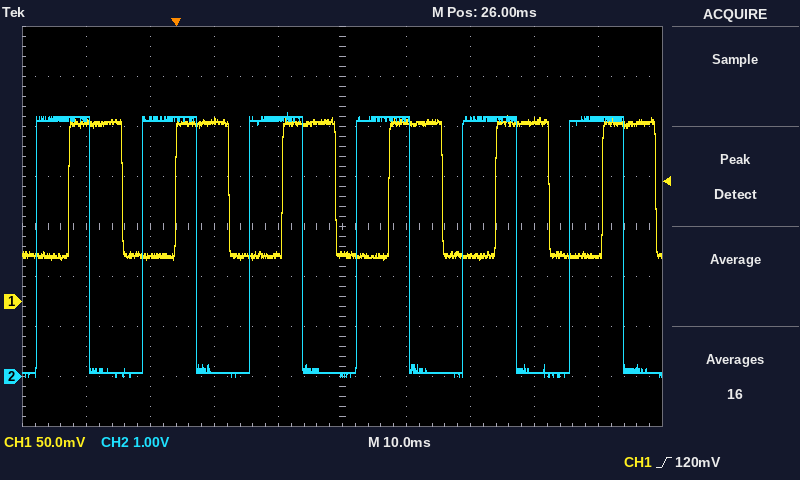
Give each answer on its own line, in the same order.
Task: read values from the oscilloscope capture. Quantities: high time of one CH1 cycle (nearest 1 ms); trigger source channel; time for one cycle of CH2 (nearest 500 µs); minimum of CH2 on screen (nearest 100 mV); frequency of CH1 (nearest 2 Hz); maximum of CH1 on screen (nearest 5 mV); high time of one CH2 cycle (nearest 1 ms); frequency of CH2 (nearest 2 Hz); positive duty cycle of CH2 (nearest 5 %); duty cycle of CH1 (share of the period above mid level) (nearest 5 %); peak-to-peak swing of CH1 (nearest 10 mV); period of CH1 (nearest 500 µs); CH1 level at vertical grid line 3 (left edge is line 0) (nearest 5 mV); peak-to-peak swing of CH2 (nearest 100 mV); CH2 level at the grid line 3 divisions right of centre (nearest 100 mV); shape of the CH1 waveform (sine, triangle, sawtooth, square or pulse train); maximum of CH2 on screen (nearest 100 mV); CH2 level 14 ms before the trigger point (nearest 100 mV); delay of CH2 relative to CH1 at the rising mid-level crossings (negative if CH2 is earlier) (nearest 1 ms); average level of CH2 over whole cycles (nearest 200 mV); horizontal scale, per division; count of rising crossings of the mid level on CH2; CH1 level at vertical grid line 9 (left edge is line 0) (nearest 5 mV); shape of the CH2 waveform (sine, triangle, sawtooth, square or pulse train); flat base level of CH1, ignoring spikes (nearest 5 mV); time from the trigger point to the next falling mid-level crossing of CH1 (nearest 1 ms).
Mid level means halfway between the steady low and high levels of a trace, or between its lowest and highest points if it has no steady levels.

8 ms
CH1
16.5 ms
0.0 V
60 Hz
185 mV
8 ms
60 Hz
50 %
50 %
140 mV
16.5 ms
180 mV
5.3 V
100 mV
square
5.3 V
5.2 V
-5 ms
2.6 V
10 ms
6
45 mV
square
45 mV
8 ms
